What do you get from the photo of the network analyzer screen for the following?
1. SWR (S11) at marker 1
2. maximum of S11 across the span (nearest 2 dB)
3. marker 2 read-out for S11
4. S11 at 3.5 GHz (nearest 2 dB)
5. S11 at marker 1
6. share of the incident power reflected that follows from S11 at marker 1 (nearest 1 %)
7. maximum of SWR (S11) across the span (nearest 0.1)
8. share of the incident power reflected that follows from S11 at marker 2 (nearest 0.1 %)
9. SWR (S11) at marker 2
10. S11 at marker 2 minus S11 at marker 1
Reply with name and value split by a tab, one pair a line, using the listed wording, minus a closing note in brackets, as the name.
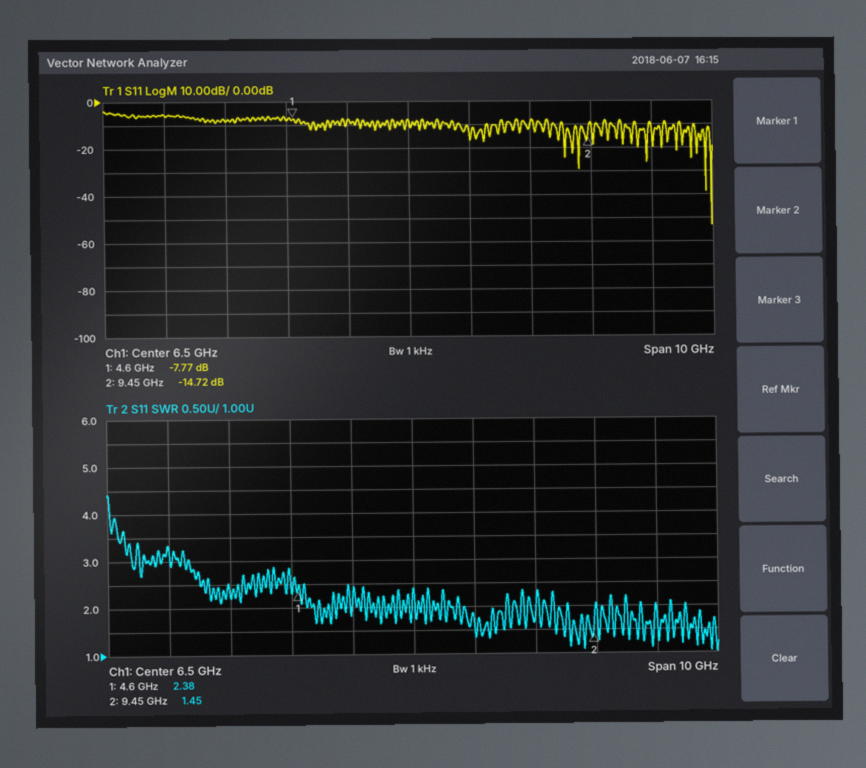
SWR (S11) at marker 1	2.38
maximum of S11 across the span	-4 dB
marker 2 read-out for S11	-14.72 dB
S11 at 3.5 GHz	-8 dB
S11 at marker 1	-7.77 dB
share of the incident power reflected that follows from S11 at marker 1	17 %
maximum of SWR (S11) across the span	4.4
share of the incident power reflected that follows from S11 at marker 2	3.4 %
SWR (S11) at marker 2	1.45
S11 at marker 2 minus S11 at marker 1	-6.95 dB
